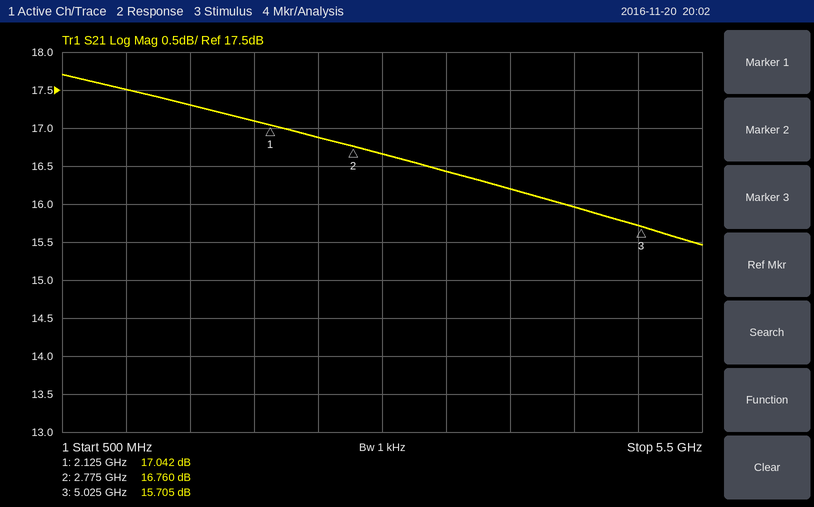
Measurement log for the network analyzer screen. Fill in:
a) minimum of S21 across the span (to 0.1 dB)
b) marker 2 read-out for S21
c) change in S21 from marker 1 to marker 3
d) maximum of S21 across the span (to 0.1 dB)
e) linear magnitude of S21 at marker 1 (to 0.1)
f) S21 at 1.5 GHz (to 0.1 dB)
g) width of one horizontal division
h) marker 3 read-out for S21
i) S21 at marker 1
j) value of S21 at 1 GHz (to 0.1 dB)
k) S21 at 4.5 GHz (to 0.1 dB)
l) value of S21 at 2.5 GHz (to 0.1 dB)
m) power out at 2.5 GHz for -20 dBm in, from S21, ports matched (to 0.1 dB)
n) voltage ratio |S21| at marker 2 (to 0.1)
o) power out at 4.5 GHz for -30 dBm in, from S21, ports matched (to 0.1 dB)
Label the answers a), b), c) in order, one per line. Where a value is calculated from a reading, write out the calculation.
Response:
a) 15.5 dB
b) 16.760 dB
c) 15.705 − (17.042) = -1.337 dB
d) 17.7 dB
e) 10^(17.042/20) ≈ 7.1
f) 17.3 dB
g) 500 MHz
h) 15.705 dB
i) 17.042 dB
j) 17.5 dB
k) 16.0 dB
l) 16.9 dB
m) -20 dBm + (16.9 dB) = -3.1 dBm
n) 10^(16.76/20) ≈ 6.9
o) -30 dBm + (16.0 dB) = -14.0 dBm
